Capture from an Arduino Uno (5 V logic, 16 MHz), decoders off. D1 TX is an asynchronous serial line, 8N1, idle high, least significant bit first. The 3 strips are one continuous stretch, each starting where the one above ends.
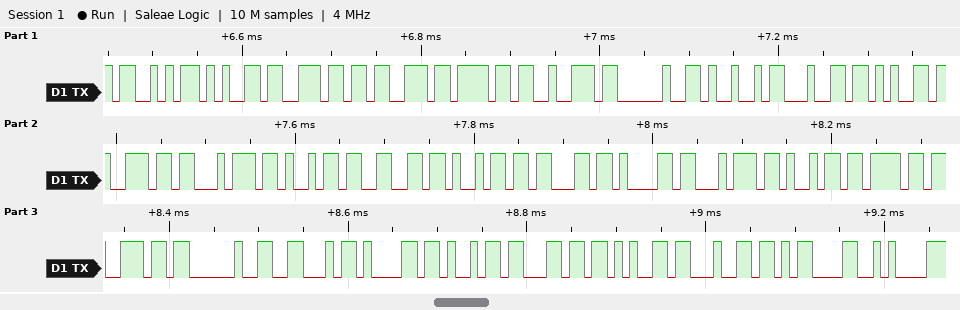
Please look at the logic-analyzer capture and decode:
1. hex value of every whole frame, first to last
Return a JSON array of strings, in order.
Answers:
["0x53 0x65 0x6E 0x73 0x6F 0x72 0x20 0x49 0x64 0x65 0x6E 0x74 0x69 0x66 0x69 0x63 0x61 0x74 0x69 0x6F 0x6E 0x20 0x46 0x61 0x69 0x6C 0x65 0x64 0x0D 0x0A"]
